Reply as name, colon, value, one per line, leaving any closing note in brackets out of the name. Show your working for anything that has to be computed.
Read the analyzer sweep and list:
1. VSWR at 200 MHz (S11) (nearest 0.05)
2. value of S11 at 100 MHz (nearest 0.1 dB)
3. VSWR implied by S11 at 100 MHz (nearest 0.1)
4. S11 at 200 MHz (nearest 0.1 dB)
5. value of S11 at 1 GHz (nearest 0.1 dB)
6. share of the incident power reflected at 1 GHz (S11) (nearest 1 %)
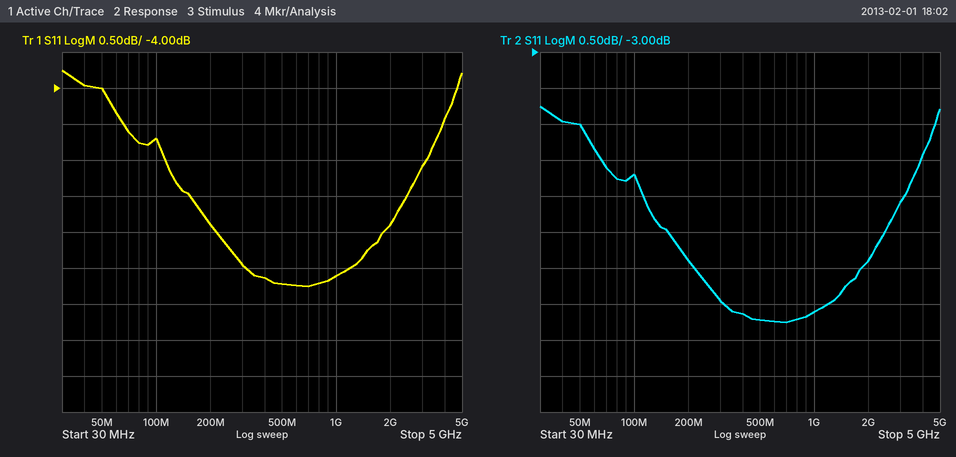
VSWR at 200 MHz (S11): |Γ| = 10^(-5.9/20) = 0.5070; VSWR = (1 + 0.5070)/(1 − 0.5070) ≈ 3.06, so 3.05 to the nearest 0.05
value of S11 at 100 MHz: -4.7 dB
VSWR implied by S11 at 100 MHz: |Γ| = 10^(-4.7/20) = 0.5821; VSWR = (1 + 0.5821)/(1 − 0.5821) ≈ 3.8
S11 at 200 MHz: -5.9 dB
value of S11 at 1 GHz: -6.6 dB
share of the incident power reflected at 1 GHz (S11): 10^(-6.6/10) ≈ 22 %
